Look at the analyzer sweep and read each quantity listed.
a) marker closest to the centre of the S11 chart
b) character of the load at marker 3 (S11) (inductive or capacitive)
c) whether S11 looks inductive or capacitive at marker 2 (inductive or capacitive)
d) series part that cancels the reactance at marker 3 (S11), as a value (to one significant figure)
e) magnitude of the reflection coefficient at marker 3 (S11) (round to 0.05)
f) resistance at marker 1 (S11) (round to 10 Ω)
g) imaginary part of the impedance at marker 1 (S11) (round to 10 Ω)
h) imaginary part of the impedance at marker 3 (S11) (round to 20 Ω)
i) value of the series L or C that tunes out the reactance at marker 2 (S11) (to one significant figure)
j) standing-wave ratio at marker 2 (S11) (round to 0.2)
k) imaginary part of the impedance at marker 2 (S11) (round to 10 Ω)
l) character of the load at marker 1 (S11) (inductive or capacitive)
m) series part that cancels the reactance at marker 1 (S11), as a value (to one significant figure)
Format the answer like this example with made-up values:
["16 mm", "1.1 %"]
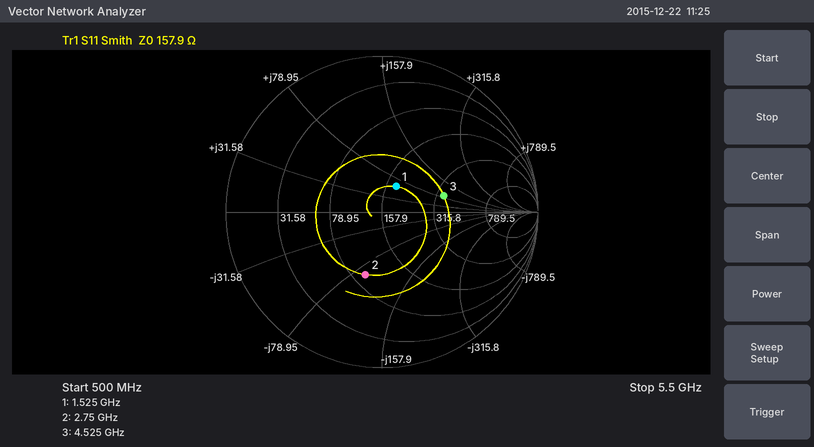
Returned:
["marker 1", "inductive", "capacitive", "400 fF", "0.40", "180 Ω", "+60 Ω", "+80 Ω", "5 nH", "2.4", "-90 Ω", "inductive", "2 pF"]
